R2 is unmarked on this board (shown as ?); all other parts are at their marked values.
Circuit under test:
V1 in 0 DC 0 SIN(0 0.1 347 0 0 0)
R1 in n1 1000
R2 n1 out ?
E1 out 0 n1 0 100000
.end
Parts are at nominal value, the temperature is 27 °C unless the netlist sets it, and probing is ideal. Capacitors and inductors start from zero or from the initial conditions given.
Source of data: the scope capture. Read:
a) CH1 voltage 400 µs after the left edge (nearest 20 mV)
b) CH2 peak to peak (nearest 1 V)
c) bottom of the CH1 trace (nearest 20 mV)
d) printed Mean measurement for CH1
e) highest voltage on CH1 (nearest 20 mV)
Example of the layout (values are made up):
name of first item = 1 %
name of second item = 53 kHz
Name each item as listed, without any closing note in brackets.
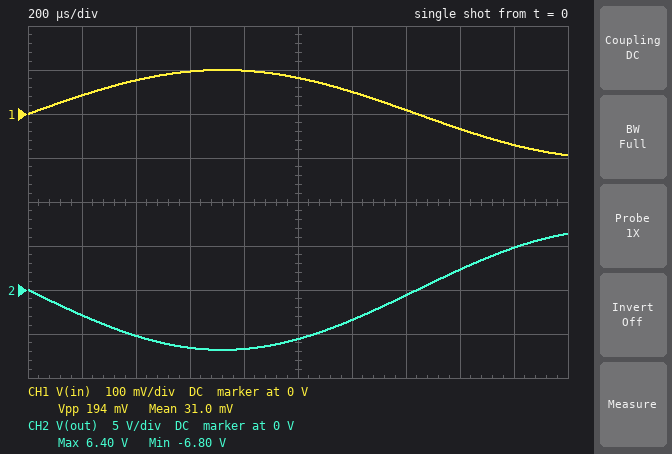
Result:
CH1 voltage 400 µs after the left edge = 80 mV
CH2 peak to peak = 13 V
bottom of the CH1 trace = -100 mV
printed Mean measurement for CH1 = 31.0 mV
highest voltage on CH1 = 100 mV
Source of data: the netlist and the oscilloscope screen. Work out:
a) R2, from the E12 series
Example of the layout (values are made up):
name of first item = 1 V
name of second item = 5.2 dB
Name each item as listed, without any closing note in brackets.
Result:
R2, from the E12 series = 68 kΩ
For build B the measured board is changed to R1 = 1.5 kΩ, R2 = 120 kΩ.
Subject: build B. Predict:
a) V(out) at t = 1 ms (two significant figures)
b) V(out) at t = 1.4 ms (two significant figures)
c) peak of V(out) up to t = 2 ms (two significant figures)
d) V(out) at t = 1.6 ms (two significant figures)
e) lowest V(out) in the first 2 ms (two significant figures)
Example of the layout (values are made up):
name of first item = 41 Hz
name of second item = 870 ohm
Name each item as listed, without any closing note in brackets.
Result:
V(out) at t = 1 ms = -6.6 V
V(out) at t = 1.4 ms = -710 mV
peak of V(out) up to t = 2 ms = 7.5 V
V(out) at t = 1.6 ms = 2.7 V
lowest V(out) in the first 2 ms = -8.0 V
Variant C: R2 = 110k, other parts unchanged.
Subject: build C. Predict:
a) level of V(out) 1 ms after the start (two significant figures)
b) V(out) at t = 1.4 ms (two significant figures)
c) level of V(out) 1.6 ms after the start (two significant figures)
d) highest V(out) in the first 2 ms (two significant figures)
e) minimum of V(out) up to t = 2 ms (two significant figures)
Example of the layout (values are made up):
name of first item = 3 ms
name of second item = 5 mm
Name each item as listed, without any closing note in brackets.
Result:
level of V(out) 1 ms after the start = -9.0 V
V(out) at t = 1.4 ms = -980 mV
level of V(out) 1.6 ms after the start = 3.7 V
highest V(out) in the first 2 ms = 10 V
minimum of V(out) up to t = 2 ms = -11 V
